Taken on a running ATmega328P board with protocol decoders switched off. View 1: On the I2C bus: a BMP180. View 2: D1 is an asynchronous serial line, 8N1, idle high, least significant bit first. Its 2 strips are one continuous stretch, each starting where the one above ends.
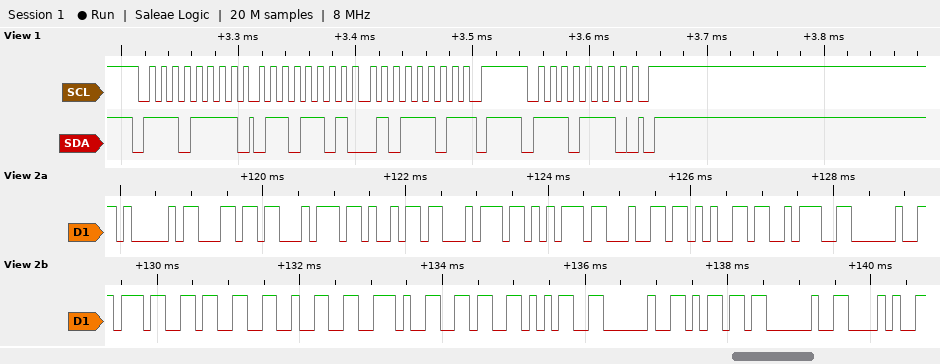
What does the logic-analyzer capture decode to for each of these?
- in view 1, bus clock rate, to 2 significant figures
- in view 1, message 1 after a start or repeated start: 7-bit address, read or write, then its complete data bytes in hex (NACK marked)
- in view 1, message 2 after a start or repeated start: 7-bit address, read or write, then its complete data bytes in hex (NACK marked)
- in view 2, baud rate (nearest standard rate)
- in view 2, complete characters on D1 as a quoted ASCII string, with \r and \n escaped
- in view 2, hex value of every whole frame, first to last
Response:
100 kHz
0x77 read: 6D 5D NACK
0x77 write
9600 baud
"Altitude: 732.65 m ("
0x41 0x6C 0x74 0x69 0x74 0x75 0x64 0x65 0x3A 0x20 0x37 0x33 0x32 0x2E 0x36 0x35 0x20 0x6D 0x20 0x28
